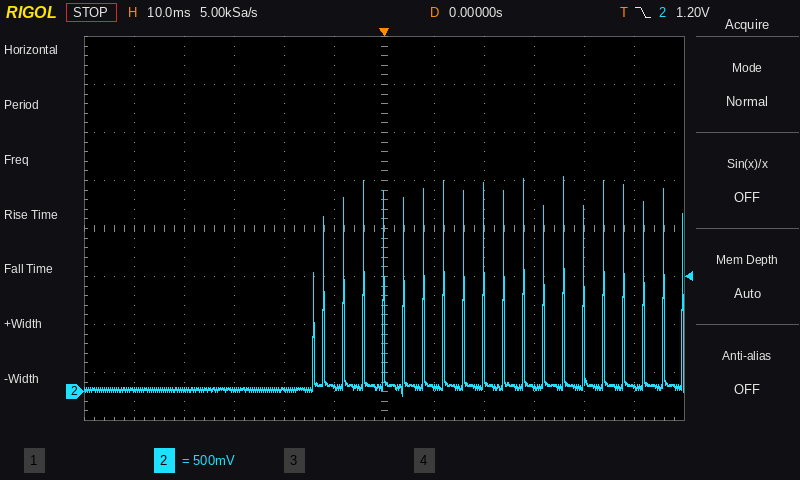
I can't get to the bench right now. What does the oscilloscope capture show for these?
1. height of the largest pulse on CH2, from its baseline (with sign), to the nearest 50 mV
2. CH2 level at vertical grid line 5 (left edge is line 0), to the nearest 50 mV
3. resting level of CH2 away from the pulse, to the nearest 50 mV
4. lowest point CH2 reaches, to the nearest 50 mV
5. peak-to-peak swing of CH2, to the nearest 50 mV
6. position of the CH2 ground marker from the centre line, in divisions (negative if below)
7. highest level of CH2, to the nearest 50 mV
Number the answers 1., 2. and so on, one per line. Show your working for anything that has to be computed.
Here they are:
1. 2.25 V − (50 mV) = +2.20 V
2. 50 mV
3. 50 mV
4. -50 mV
5. 2.25 V − (-50 mV) = 2.30 V
6. -3.4 div
7. 2.25 V
